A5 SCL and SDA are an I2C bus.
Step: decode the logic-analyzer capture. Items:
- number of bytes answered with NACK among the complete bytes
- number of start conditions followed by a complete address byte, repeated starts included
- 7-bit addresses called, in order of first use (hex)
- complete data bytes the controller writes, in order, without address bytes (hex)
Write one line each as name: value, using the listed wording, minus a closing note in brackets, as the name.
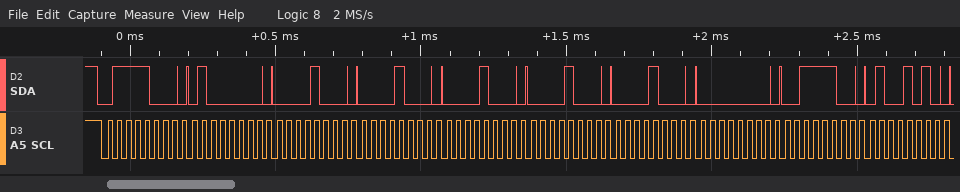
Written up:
number of bytes answered with NACK among the complete bytes: 0
number of start conditions followed by a complete address byte, repeated starts included: 1
7-bit addresses called, in order of first use: 0x3C
complete data bytes the controller writes, in order, without address bytes: 40 08 08 08 08 08 00 3C 4A
